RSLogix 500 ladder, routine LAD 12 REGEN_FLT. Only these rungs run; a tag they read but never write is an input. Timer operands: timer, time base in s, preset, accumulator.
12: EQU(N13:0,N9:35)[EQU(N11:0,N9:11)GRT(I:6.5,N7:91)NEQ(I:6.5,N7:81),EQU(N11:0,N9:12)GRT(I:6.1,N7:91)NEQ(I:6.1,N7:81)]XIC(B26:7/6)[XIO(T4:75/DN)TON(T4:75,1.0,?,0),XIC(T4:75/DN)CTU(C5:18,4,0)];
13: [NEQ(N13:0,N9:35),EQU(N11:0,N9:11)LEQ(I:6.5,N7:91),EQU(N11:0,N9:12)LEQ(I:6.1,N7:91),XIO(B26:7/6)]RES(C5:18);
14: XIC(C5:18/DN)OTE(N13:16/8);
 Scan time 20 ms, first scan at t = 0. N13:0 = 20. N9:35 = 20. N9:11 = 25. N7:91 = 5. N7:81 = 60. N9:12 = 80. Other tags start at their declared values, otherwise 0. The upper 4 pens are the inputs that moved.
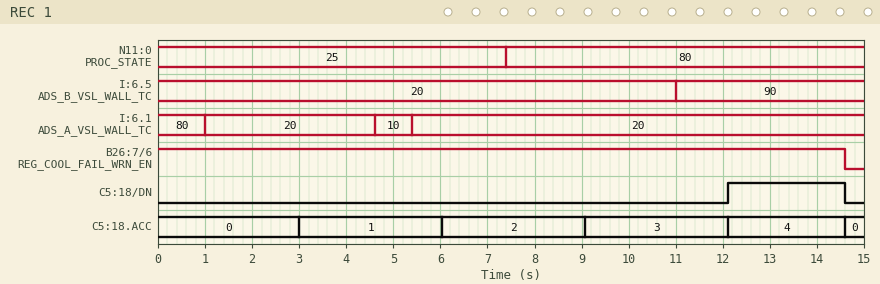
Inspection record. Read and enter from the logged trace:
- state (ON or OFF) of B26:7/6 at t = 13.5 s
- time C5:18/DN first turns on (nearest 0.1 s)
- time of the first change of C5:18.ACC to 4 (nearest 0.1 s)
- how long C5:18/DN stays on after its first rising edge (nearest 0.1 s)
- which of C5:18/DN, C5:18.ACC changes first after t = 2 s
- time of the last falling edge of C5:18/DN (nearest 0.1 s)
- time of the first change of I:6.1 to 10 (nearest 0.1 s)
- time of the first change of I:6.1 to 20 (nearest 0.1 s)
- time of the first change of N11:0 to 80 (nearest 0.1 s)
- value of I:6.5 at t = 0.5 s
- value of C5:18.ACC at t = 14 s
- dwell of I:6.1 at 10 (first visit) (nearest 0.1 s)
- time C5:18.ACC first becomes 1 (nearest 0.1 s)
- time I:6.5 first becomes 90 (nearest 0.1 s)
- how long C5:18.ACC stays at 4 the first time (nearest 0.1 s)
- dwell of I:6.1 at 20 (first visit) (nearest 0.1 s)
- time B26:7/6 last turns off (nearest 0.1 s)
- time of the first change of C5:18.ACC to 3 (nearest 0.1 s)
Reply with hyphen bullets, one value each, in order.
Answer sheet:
- ON
- 12.1 s
- 12.1 s
- 2.5 s
- C5:18.ACC
- 14.6 s
- 4.6 s
- 1.0 s
- 7.4 s
- 20
- 4
- 0.8 s
- 3.0 s
- 11.0 s
- 2.5 s
- 3.6 s
- 14.6 s
- 9.1 s
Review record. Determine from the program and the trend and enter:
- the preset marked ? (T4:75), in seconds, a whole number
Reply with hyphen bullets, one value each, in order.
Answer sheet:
- 3 s
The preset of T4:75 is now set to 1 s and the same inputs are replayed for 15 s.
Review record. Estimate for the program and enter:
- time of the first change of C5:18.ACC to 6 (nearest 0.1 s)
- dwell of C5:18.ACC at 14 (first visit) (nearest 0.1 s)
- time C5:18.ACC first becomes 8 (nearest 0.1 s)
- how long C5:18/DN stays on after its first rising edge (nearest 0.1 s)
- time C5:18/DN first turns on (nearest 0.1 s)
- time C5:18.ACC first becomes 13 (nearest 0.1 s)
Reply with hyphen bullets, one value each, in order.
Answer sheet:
- 6.2 s
- 0.1 s
- 8.3 s
- 10.5 s
- 4.1 s
- 13.5 s
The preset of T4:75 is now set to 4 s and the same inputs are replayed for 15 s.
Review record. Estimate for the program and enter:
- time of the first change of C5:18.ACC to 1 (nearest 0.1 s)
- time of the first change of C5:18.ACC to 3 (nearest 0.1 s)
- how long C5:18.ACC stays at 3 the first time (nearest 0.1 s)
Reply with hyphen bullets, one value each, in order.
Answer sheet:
- 4.0 s
- 12.1 s
- 2.5 s
